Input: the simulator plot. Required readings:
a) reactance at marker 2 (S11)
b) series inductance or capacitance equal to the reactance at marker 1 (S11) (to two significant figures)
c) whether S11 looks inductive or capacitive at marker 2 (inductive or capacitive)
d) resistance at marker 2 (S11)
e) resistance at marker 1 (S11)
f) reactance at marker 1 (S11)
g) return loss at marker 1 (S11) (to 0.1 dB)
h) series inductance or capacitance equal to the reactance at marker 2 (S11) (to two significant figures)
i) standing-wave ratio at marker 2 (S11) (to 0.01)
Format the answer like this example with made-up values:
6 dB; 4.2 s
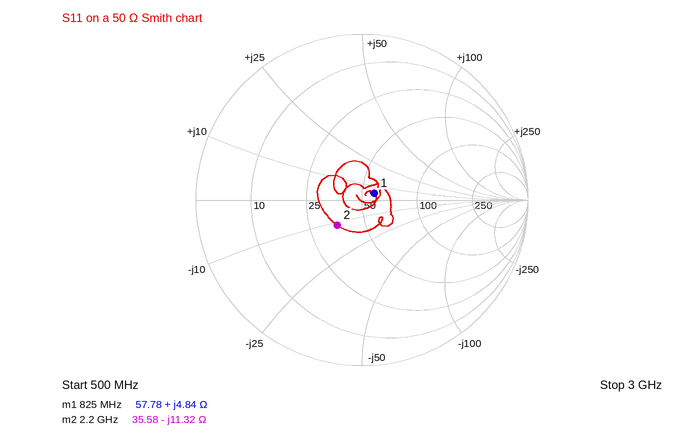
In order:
-11.32 Ω; 930 pH; capacitive; 35.58 Ω; 57.78 Ω; +4.84 Ω; 21.4 dB; 6.4 pF; 1.54
